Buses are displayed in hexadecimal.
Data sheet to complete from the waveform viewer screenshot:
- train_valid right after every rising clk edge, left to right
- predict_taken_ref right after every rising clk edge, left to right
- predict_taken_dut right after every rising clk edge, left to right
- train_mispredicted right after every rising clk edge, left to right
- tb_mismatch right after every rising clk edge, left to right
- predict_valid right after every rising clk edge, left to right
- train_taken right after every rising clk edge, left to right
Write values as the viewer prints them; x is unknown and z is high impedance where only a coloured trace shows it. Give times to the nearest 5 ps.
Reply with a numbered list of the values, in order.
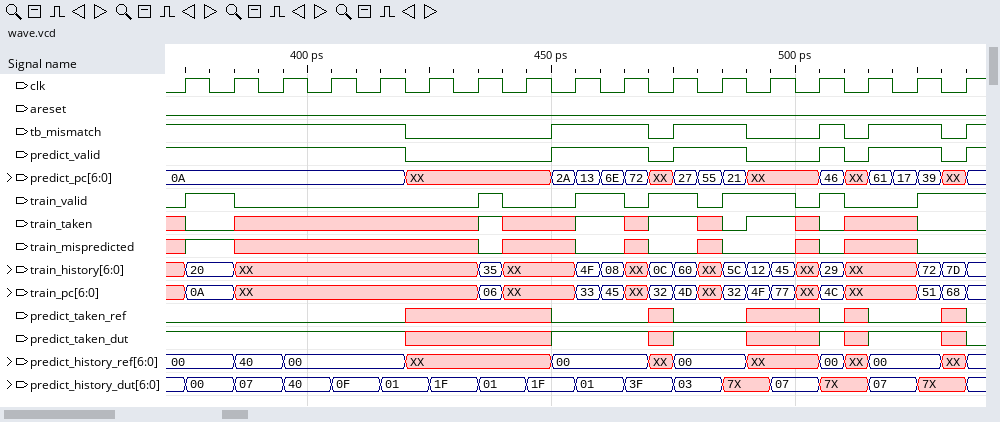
1. 1 0 0 0 0 0 1 0 1 0 1 1 1 1 0 1 1
2. 0 0 0 0 0 x x x 0 0 0 0 x 0 0 0 0
3. 1 1 1 1 1 x x x 1 1 1 1 x 1 1 1 0
4. 1 x x x x x 0 x 0 x 0 0 0 0 x 0 0
5. 1 1 1 1 1 0 0 0 1 1 1 1 0 1 1 1 1
6. 1 1 1 1 1 0 0 0 1 1 1 1 0 1 1 1 1
7. 0 x x x x x 1 x 1 x 1 0 1 0 x 0 0
